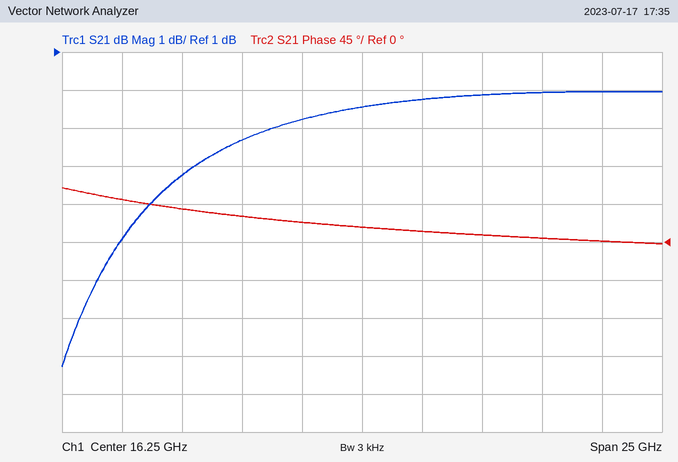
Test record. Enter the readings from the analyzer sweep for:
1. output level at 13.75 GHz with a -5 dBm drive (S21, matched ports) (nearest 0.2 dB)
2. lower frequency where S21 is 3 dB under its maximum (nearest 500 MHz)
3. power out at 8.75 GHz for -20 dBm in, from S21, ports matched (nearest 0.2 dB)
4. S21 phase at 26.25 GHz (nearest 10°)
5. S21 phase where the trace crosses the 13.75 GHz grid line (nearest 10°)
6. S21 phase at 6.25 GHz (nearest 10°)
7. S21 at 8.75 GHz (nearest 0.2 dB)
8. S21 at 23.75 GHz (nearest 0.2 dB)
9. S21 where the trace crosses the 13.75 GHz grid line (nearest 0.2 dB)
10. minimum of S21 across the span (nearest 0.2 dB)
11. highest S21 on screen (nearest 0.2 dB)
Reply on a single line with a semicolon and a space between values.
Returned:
-5.8 dBm; 7.5 GHz; -22.2 dBm; 0°; 20°; 50°; -2.2 dB; 0.0 dB; -0.8 dB; -7.2 dB; 0.0 dB
